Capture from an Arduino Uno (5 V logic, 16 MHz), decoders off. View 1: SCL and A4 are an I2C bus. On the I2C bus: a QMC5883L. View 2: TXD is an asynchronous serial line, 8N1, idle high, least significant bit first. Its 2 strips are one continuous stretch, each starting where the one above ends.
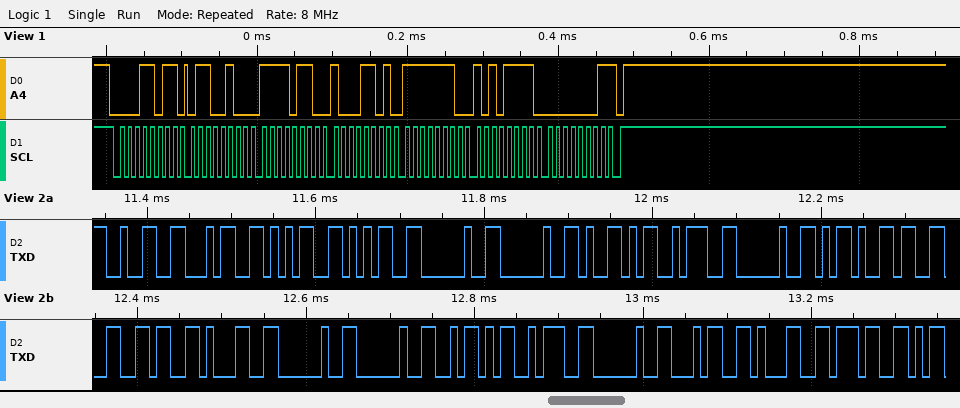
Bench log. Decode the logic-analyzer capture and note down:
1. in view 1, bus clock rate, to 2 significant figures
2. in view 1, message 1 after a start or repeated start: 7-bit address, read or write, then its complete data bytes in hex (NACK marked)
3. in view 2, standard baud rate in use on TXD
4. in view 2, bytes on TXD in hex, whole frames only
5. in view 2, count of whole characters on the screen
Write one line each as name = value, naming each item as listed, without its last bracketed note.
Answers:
in view 1, bus clock rate, to 2 significant figures = 100 kHz
in view 1, message 1 after a start or repeated start: 7-bit address, read or write, then its complete data bytes in hex = 0x0D read: 64 F6 8D FE AF 01 NACK
in view 2, standard baud rate in use on TXD = 115200 baud
in view 2, bytes on TXD in hex, whole frames only = 32 34 35 35 20 20 59 3A 20 2D 33 36 31 20 20 5A 3A 20 34 31 37
in view 2, count of whole characters on the screen = 21
